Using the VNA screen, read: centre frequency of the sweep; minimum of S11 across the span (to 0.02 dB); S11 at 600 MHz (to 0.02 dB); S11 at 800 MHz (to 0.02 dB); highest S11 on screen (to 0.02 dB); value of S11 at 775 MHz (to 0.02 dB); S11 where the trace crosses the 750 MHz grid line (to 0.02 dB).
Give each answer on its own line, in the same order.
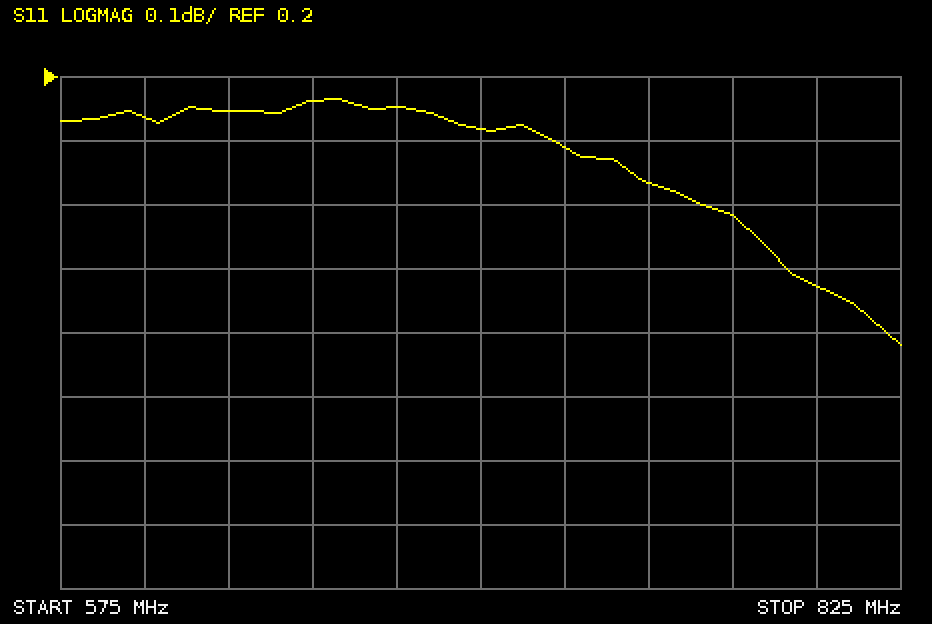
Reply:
700 MHz
-0.22 dB
0.14 dB
-0.12 dB
0.16 dB
-0.02 dB
0.04 dB
